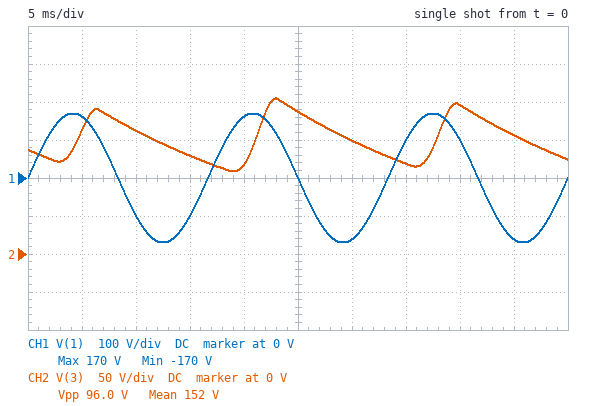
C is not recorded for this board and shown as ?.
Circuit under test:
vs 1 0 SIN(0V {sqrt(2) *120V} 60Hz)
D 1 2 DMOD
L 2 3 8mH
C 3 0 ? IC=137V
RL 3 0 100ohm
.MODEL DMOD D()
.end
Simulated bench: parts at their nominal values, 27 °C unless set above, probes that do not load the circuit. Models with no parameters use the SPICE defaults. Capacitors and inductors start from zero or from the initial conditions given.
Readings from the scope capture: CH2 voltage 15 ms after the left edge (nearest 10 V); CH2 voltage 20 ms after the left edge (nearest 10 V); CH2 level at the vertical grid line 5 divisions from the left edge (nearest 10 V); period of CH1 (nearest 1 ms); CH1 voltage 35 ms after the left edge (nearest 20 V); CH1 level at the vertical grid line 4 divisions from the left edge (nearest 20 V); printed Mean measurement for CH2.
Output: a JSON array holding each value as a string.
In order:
["130 V", "120 V", "190 V", "17 ms", "100 V", "160 V", "152 V"]
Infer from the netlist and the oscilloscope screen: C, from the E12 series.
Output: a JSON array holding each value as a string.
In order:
["220 µF"]
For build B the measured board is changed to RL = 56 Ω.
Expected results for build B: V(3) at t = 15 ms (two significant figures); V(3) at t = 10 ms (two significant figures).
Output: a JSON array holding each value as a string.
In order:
["99 V", "150 V"]
